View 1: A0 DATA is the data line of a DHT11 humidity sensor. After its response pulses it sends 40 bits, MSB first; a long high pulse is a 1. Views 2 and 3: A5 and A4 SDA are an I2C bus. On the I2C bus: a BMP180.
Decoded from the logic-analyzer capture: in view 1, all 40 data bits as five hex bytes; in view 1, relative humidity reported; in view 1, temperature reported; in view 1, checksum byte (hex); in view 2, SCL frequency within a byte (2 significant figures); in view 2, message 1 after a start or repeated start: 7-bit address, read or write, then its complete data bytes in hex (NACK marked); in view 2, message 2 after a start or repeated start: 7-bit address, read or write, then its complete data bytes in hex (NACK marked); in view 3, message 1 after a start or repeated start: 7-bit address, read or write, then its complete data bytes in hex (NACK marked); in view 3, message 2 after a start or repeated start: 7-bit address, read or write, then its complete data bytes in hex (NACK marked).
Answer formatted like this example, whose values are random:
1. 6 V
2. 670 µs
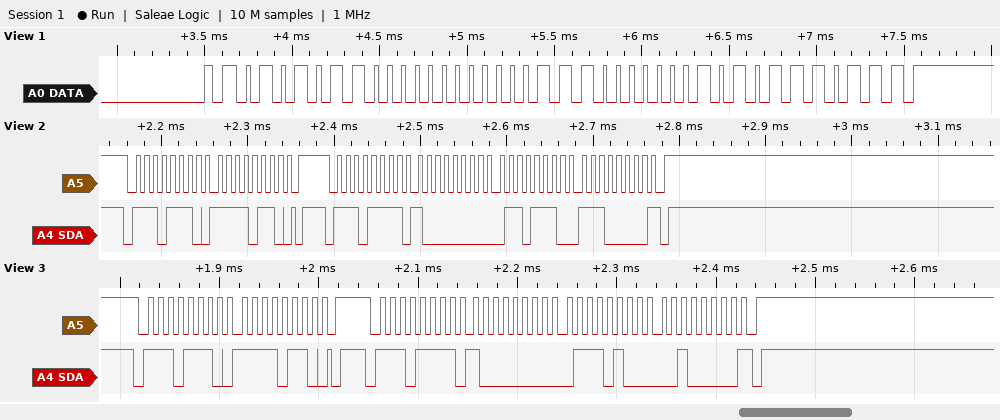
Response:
1. 56 00 1C 05 77
2. 86 %
3. 28.5 °C
4. 0x77
5. 100 kHz
6. 0x77 write: F6
7. 0x77 read: 80 6E E0 NACK
8. 0x77 write: F6
9. 0x77 read: 80 74 20 NACK
